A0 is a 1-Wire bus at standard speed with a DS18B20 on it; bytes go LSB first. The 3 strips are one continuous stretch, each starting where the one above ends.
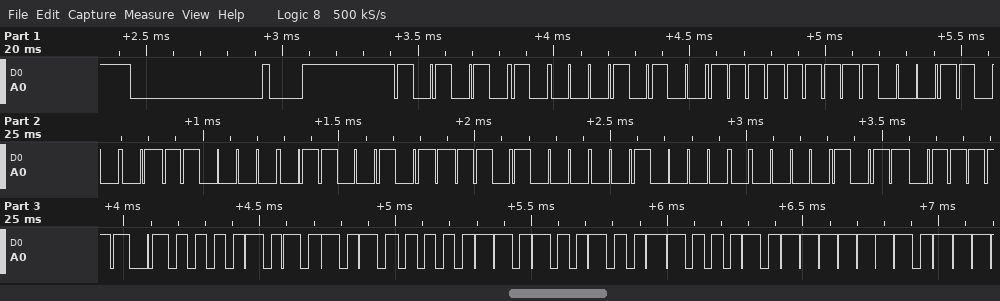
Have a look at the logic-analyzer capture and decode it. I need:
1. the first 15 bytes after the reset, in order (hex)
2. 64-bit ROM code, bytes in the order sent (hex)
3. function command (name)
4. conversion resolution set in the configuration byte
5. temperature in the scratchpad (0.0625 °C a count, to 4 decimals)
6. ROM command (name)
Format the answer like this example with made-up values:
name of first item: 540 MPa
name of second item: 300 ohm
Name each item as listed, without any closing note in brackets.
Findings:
the first 15 bytes after the reset, in order: 55 28 FF 31 0E A6 17 04 D0 BE 50 05 4B 46 7F
64-bit ROM code, bytes in the order sent: 28 FF 31 0E A6 17 04 D0
function command: Read Scratchpad
conversion resolution set in the configuration byte: 12 bits
temperature in the scratchpad: 85.0000 °C
ROM command: Match ROM
